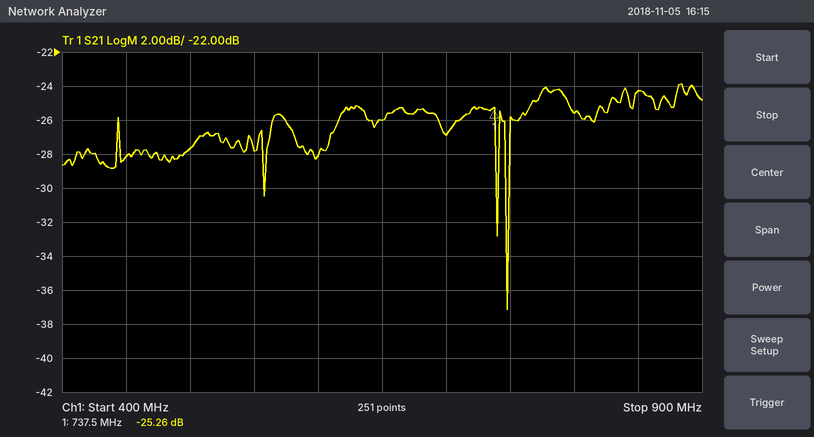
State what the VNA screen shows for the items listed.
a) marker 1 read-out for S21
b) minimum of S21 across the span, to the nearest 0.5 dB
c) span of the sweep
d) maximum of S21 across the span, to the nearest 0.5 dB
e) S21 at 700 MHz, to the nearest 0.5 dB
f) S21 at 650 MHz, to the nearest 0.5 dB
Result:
-25.26 dB
-37.0 dB
500 MHz
-24.0 dB
-27.0 dB
-26.0 dB
